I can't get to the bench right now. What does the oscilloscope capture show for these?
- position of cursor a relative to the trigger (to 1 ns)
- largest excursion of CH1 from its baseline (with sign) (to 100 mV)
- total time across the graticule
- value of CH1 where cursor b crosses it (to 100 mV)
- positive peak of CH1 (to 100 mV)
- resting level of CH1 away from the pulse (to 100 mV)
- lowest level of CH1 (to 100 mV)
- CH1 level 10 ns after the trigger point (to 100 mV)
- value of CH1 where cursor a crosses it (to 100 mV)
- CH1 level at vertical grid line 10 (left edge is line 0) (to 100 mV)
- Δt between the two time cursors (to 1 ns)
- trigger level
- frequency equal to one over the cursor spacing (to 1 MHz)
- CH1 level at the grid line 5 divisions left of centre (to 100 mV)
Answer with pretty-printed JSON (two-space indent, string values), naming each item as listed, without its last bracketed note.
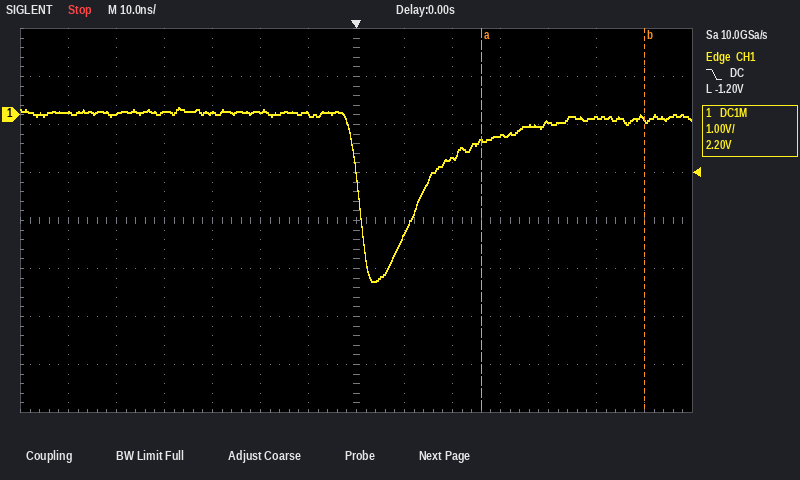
{
  "position of cursor a relative to the trigger": "+26 ns",
  "largest excursion of CH1 from its baseline (with sign)": "-3.5 V",
  "total time across the graticule": "140 ns",
  "value of CH1 where cursor b crosses it": "-100 mV",
  "positive peak of CH1": "200 mV",
  "resting level of CH1 away from the pulse": "0.0 V",
  "lowest level of CH1": "-3.5 V",
  "CH1 level 10 ns after the trigger point": "-2.5 V",
  "value of CH1 where cursor a crosses it": "-600 mV",
  "CH1 level at vertical grid line 10 (left edge is line 0)": "-400 mV",
  "Δt between the two time cursors": "34 ns",
  "trigger level": "-1.20 V",
  "frequency equal to one over the cursor spacing": "29 MHz",
  "CH1 level at the grid line 5 divisions left of centre": "0.0 V"
}
